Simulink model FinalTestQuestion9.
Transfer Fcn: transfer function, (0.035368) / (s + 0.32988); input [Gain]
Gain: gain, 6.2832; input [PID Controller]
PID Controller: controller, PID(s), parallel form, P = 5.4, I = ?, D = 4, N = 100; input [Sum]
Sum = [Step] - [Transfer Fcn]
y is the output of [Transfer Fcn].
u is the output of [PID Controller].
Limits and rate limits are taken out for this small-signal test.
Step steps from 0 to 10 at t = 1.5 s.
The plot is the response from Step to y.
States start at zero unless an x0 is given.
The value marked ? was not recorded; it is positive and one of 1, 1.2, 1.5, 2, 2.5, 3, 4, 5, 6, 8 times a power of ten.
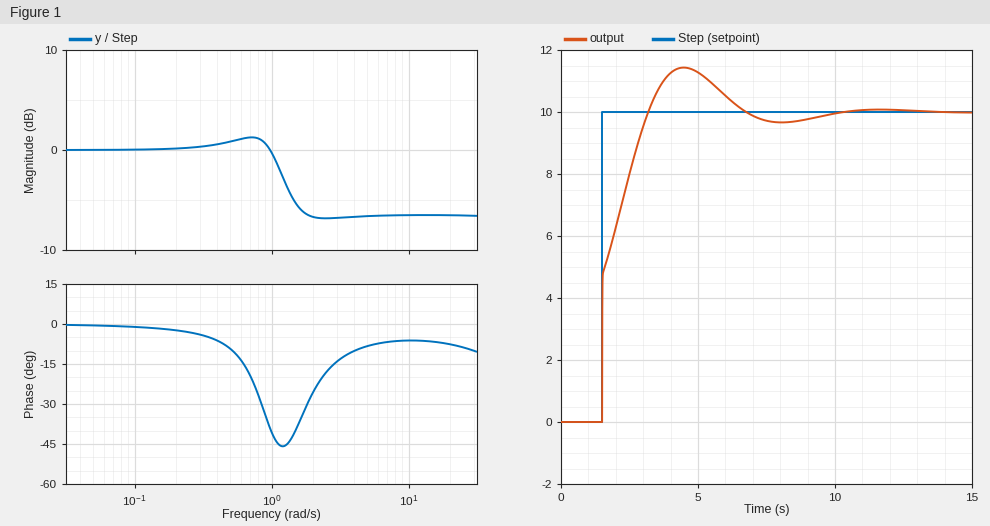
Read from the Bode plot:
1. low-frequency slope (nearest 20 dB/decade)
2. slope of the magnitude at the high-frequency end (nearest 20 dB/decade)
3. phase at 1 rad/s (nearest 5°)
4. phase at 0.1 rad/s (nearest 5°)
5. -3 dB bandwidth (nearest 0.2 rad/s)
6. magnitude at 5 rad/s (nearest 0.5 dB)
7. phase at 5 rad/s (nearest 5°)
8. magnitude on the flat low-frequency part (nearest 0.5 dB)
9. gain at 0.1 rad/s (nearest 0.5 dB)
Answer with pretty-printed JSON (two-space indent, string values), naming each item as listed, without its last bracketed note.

{
  "low-frequency slope": "0 dB/decade",
  "slope of the magnitude at the high-frequency end": "0 dB/decade",
  "phase at 1 rad/s": "-40°",
  "phase at 0.1 rad/s": "0°",
  "-3 dB bandwidth": "1.2 rad/s",
  "magnitude at 5 rad/s": "-6.5 dB",
  "phase at 5 rad/s": "-10°",
  "magnitude on the flat low-frequency part": "0.0 dB",
  "gain at 0.1 rad/s": "0.0 dB"
}
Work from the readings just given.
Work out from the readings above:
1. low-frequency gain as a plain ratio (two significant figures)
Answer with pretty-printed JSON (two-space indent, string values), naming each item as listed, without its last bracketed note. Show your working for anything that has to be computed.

{
  "low-frequency gain as a plain ratio": "10^(0 / 20) = 1.0"
}
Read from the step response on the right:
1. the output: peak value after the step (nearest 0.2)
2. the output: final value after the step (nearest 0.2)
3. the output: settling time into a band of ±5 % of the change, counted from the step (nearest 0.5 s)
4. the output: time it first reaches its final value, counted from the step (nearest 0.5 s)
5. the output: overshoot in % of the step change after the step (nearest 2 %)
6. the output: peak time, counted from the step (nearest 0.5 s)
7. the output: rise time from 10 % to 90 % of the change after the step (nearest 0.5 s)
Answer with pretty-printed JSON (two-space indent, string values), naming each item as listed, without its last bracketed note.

{
  "the output: peak value after the step": "11.4",
  "the output: final value after the step": "10.0",
  "the output: settling time into a band of ±5 % of the change, counted from the step": "4.5 s",
  "the output: time it first reaches its final value, counted from the step": "1.5 s",
  "the output: overshoot in % of the step change after the step": "14 %",
  "the output: peak time, counted from the step": "3.0 s",
  "the output: rise time from 10 % to 90 % of the change after the step": "1.5 s"
}
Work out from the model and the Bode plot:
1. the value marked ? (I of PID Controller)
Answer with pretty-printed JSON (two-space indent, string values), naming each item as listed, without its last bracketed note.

{
  "the value marked ?": "8"
}
